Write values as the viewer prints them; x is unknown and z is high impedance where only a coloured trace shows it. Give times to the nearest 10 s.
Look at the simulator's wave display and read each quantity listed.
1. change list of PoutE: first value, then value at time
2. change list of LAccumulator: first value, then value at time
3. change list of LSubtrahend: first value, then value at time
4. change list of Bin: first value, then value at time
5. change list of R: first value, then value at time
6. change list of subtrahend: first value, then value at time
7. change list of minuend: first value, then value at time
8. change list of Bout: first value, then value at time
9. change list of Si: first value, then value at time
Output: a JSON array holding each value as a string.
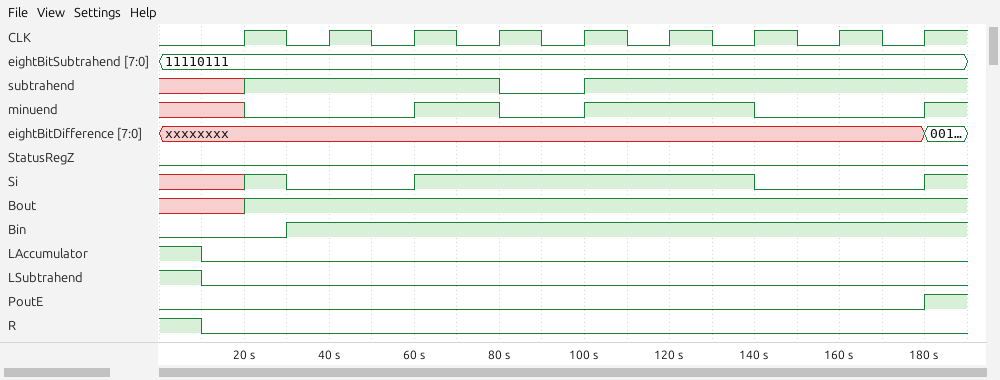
["0, 1 at 180 s", "1, 0 at 10 s", "1, 0 at 10 s", "0, 1 at 30 s", "1, 0 at 10 s", "x, 1 at 20 s, 0 at 80 s, 1 at 100 s", "x, 0 at 20 s, 1 at 60 s, 0 at 80 s, 1 at 100 s, 0 at 140 s, 1 at 180 s", "x, 1 at 20 s", "x, 1 at 20 s, 0 at 30 s, 1 at 60 s, 0 at 140 s, 1 at 180 s"]
